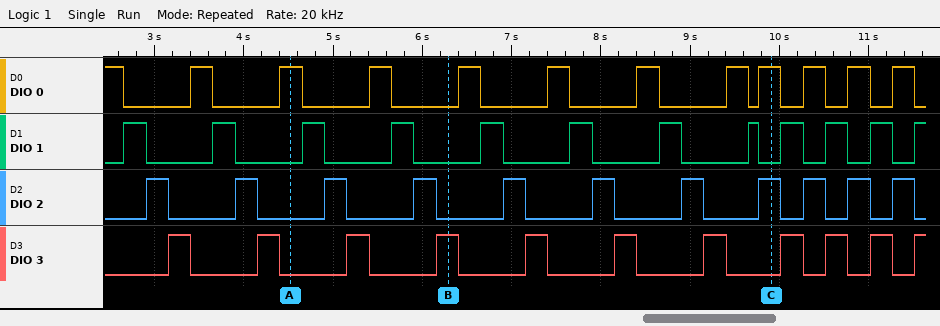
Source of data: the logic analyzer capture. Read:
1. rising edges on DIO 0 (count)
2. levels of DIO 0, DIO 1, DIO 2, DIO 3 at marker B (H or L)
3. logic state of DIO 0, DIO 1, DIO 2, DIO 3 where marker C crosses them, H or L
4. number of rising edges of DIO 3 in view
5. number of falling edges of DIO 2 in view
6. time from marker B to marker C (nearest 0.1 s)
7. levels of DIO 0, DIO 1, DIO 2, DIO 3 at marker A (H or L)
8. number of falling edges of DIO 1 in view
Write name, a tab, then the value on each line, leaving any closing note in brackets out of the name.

rising edges on DIO 0	11
levels of DIO 0, DIO 1, DIO 2, DIO 3 at marker B	DIO 0=L, DIO 1=L, DIO 2=L, DIO 3=H
logic state of DIO 0, DIO 1, DIO 2, DIO 3 where marker C crosses them, H or L	DIO 0=H, DIO 1=L, DIO 2=H, DIO 3=L
number of rising edges of DIO 3 in view	11
number of falling edges of DIO 2 in view	11
time from marker B to marker C	3.6 s
levels of DIO 0, DIO 1, DIO 2, DIO 3 at marker A	DIO 0=H, DIO 1=L, DIO 2=L, DIO 3=L
number of falling edges of DIO 1 in view	11
